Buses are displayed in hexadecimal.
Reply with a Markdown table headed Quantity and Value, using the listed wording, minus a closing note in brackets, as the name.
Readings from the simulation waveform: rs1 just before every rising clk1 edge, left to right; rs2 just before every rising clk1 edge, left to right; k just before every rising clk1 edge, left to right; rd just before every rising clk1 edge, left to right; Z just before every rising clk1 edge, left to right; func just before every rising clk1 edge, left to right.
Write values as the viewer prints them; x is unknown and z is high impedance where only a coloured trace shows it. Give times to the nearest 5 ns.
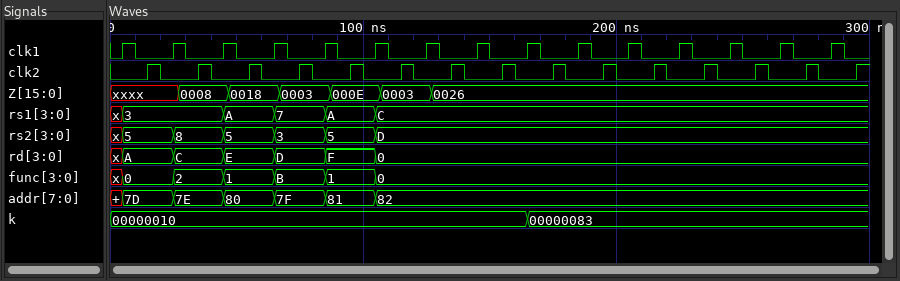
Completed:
| Quantity | Value |
|---|---|
| rs1 just before every rising clk1 edge, left to right | x, 3, 3, A, 7, A, C, C, C, C, C, C, C, C, C |
| rs2 just before every rising clk1 edge, left to right | x, 5, 8, 5, 3, 5, D, D, D, D, D, D, D, D, D |
| k just before every rising clk1 edge, left to right | 00000010, 00000010, 00000010, 00000010, 00000010, 00000010, 00000010, 00000010, 00000010, 00000083, 00000083, 00000083, 00000083, 00000083, 00000083 |
| rd just before every rising clk1 edge, left to right | x, A, C, E, D, F, 0, 0, 0, 0, 0, 0, 0, 0, 0 |
| Z just before every rising clk1 edge, left to right | xxxx, xxxx, 0008, 0018, 0003, 000E, 0003, 0026, 0026, 0026, 0026, 0026, 0026, 0026, 0026 |
| func just before every rising clk1 edge, left to right | x, 0, 2, 1, B, 1, 0, 0, 0, 0, 0, 0, 0, 0, 0 |
